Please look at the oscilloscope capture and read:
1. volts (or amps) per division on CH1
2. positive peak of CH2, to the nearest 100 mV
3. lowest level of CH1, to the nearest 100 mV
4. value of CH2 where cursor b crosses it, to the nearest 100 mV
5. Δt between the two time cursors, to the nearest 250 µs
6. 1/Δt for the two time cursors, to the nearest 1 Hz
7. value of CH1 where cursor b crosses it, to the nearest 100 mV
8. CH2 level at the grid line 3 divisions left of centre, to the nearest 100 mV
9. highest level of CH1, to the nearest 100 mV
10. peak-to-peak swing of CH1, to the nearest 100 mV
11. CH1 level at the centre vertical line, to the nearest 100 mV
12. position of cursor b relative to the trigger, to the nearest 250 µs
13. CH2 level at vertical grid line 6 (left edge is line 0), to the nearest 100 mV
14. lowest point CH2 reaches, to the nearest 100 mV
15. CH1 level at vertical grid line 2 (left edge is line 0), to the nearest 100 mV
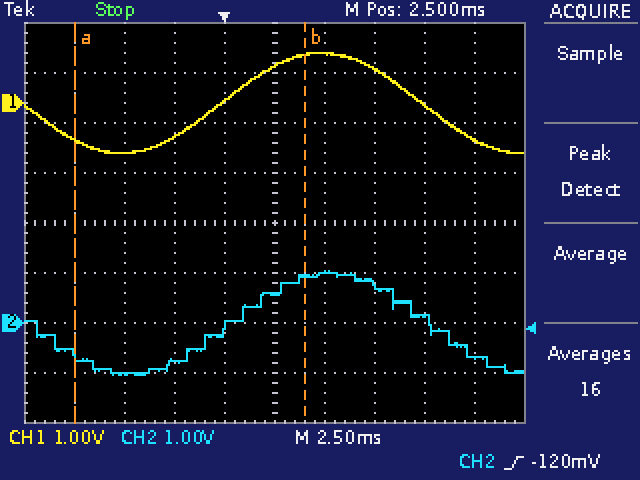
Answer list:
1 V
1.0 V
-1.0 V
900 mV
11.50 ms
87 Hz
1.0 V
-1.0 V
1.0 V
2.0 V
700 mV
+4.00 ms
1.0 V
-1.0 V
-1.0 V
